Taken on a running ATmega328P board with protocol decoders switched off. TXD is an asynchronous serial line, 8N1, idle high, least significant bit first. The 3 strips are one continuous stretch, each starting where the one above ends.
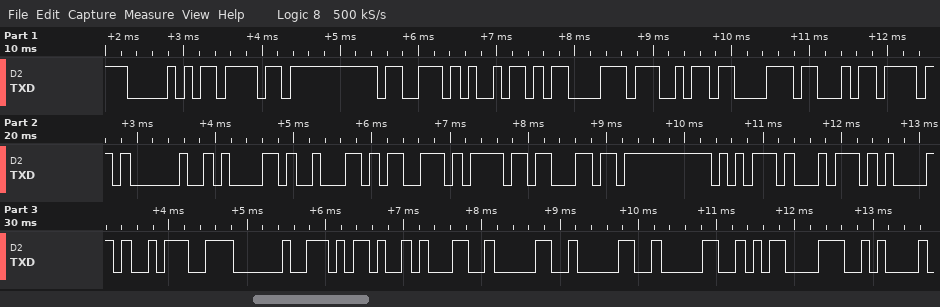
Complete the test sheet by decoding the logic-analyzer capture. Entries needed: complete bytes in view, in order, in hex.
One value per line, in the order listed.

50 6F 73 69 C3 A7 C3 A3 6F 20 61 62 73 6F 6C 75 74 61 3A 20 2D 31 30 30 30 0D 0A
